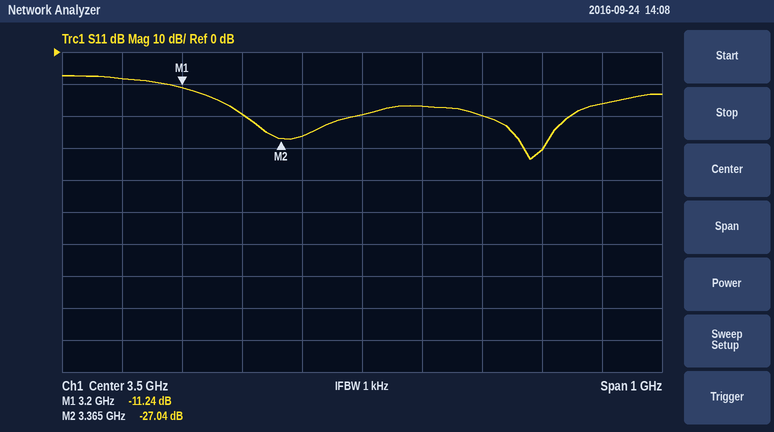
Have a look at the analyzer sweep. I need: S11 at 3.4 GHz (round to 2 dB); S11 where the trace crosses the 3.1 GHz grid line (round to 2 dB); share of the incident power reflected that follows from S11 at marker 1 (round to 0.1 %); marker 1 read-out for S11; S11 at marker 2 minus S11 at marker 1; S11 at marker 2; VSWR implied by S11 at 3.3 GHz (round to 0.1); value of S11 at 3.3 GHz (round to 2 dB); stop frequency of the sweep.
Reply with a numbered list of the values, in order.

1. -26 dB
2. -8 dB
3. 7.5 %
4. -11.24 dB
5. -15.80 dB
6. -27.04 dB
7. 1.2
8. -20 dB
9. 4 GHz
